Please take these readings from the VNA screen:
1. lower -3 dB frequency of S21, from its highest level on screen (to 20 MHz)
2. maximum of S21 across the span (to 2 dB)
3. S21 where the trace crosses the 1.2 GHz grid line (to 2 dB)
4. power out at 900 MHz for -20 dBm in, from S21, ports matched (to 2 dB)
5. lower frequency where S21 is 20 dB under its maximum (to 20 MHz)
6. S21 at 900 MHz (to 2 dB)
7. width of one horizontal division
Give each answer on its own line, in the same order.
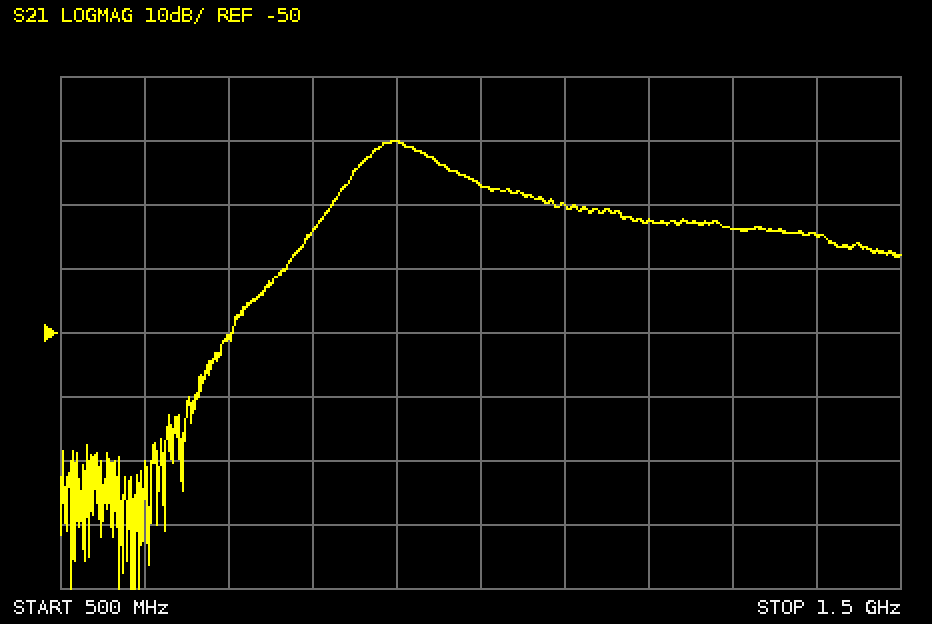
860 MHz
-20 dB
-32 dB
-40 dBm
760 MHz
-20 dB
100 MHz
